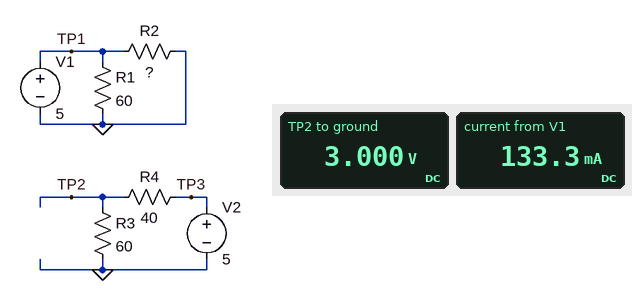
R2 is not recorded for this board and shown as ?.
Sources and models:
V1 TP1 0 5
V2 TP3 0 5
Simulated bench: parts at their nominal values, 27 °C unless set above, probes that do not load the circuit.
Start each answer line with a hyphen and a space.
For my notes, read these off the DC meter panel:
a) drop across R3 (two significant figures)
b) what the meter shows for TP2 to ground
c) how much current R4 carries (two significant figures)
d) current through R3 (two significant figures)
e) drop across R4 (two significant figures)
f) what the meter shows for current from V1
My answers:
- 3.0 V
- 3.000 V
- 50 mA
- 50 mA
- 2.0 V
- 133.3 mA
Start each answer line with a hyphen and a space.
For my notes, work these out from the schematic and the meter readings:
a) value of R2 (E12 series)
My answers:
- 100 Ω
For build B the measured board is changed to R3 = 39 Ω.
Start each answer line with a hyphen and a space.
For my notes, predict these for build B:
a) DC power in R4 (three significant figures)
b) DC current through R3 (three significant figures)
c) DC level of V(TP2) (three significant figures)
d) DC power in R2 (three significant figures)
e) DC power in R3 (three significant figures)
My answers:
- 160 mW
- 63.3 mA
- 2.47 V
- 250 mW
- 156 mW
